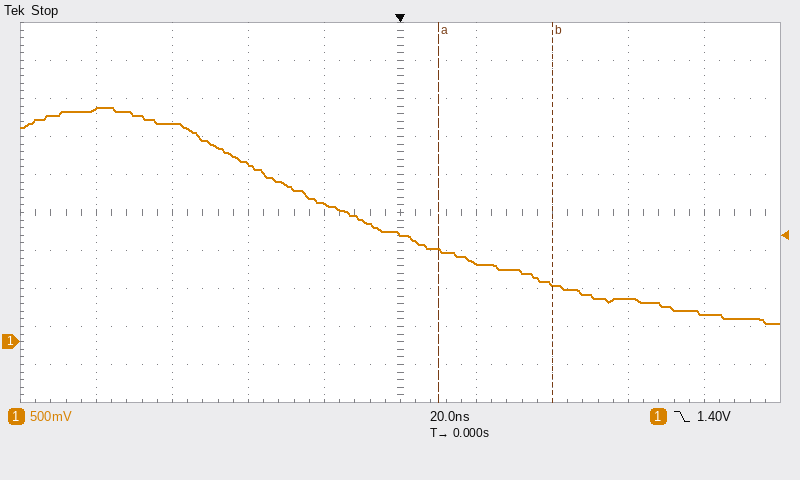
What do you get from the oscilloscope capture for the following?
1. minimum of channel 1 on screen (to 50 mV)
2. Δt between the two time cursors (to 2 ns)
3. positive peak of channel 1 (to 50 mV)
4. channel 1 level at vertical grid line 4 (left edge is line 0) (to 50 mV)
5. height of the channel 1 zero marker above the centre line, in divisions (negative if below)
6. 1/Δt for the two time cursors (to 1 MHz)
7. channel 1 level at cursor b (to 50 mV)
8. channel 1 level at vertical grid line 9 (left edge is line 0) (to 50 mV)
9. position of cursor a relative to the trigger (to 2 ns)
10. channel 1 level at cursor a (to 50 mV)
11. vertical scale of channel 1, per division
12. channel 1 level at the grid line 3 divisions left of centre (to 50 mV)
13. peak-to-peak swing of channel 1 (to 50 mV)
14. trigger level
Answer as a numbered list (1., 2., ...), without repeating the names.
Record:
1. 250 mV
2. 30 ns
3. 3.10 V
4. 1.80 V
5. -3.4 div
6. 33 MHz
7. 750 mV
8. 350 mV
9. +10 ns
10. 1.20 V
11. 500 mV
12. 2.85 V
13. 2.85 V
14. 1.40 V
